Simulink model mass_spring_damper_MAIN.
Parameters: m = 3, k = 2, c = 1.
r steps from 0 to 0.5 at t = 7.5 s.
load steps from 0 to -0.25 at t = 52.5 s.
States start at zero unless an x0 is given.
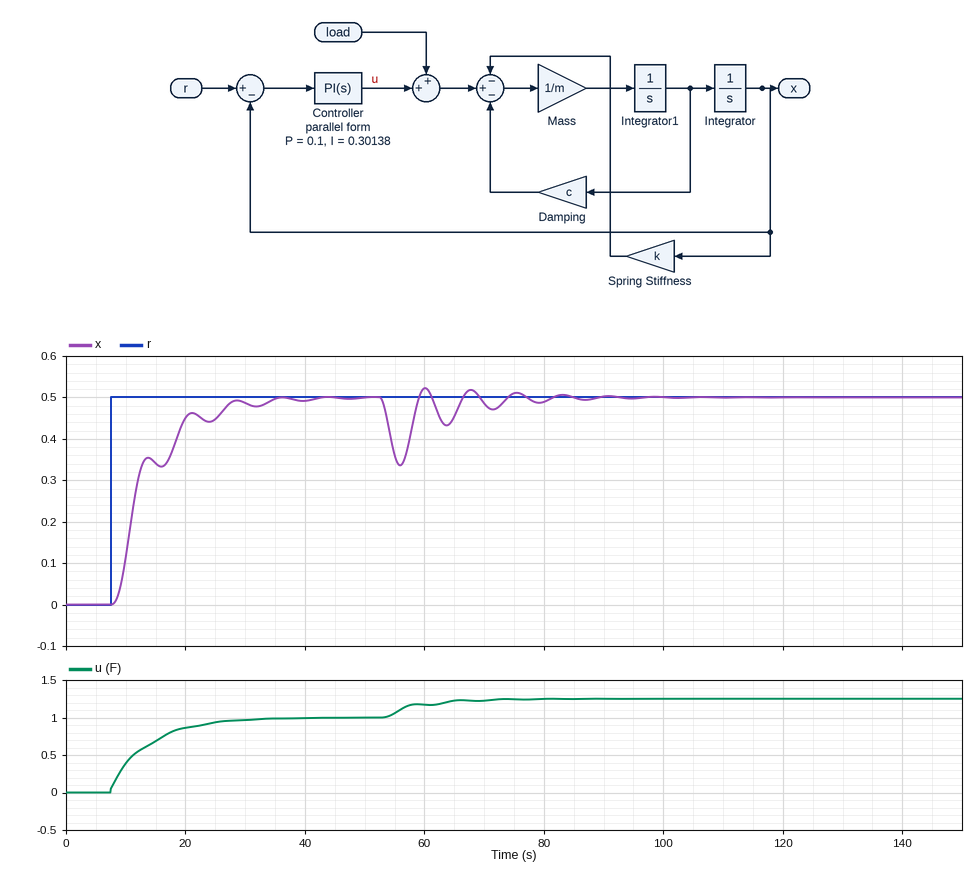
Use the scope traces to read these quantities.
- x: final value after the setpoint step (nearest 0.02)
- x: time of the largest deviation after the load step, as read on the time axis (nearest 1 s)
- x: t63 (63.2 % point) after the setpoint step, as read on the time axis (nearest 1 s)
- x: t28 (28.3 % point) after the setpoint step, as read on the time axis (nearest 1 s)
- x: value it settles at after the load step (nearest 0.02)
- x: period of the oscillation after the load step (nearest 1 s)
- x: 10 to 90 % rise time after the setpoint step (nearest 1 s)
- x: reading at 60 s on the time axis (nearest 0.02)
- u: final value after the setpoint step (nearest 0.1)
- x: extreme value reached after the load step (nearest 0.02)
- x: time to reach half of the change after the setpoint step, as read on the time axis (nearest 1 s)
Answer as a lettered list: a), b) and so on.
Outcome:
a) 0.50
b) 56 s
c) 12 s
d) 10 s
e) 0.50
f) 8 s
g) 11 s
h) 0.52
i) 1.0
j) 0.34
k) 11 s
